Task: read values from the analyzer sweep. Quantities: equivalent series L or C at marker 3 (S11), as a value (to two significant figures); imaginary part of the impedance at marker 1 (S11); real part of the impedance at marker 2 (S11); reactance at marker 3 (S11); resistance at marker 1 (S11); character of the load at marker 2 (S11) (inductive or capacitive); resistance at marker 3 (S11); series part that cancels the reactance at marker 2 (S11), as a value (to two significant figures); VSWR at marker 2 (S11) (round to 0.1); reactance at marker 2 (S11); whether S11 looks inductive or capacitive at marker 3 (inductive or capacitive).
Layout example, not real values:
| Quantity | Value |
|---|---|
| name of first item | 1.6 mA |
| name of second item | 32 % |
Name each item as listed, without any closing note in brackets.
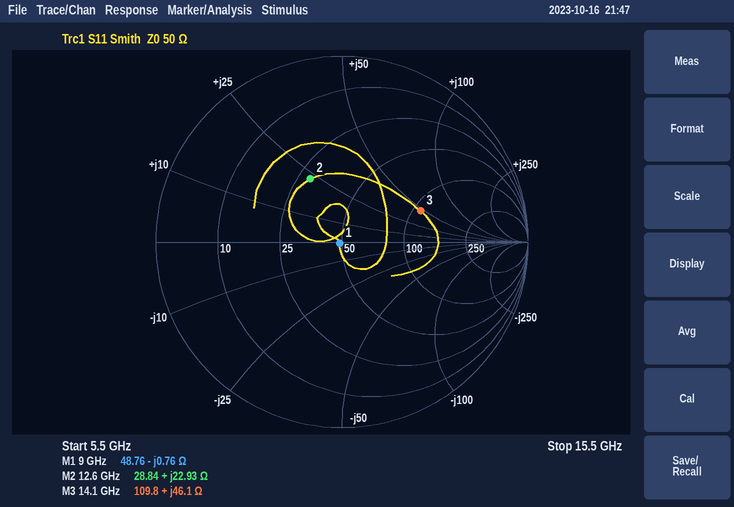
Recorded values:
| Quantity | Value |
|---|---|
| equivalent series L or C at marker 3 (S11), as a value | 520 pH |
| imaginary part of the impedance at marker 1 | -0.76 Ω |
| real part of the impedance at marker 2 | 28.84 Ω |
| reactance at marker 3 | +46.1 Ω |
| resistance at marker 1 | 48.76 Ω |
| character of the load at marker 2 (S11) | inductive |
| resistance at marker 3 | 109.8 Ω |
| series part that cancels the reactance at marker 2 (S11), as a value | 550 fF |
| VSWR at marker 2 (S11) | 2.2 |
| reactance at marker 2 | +22.93 Ω |
| whether S11 looks inductive or capacitive at marker 3 | inductive |
